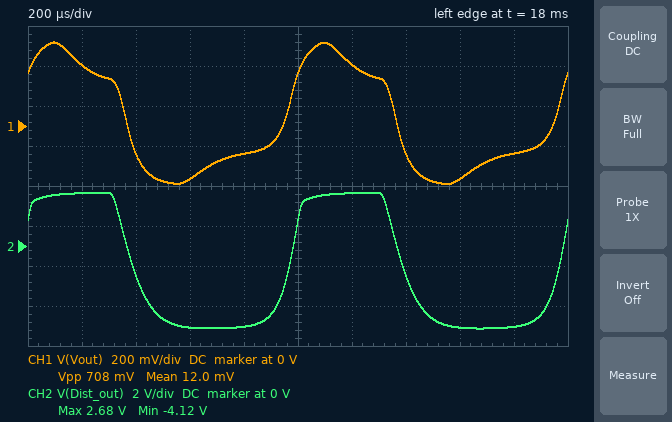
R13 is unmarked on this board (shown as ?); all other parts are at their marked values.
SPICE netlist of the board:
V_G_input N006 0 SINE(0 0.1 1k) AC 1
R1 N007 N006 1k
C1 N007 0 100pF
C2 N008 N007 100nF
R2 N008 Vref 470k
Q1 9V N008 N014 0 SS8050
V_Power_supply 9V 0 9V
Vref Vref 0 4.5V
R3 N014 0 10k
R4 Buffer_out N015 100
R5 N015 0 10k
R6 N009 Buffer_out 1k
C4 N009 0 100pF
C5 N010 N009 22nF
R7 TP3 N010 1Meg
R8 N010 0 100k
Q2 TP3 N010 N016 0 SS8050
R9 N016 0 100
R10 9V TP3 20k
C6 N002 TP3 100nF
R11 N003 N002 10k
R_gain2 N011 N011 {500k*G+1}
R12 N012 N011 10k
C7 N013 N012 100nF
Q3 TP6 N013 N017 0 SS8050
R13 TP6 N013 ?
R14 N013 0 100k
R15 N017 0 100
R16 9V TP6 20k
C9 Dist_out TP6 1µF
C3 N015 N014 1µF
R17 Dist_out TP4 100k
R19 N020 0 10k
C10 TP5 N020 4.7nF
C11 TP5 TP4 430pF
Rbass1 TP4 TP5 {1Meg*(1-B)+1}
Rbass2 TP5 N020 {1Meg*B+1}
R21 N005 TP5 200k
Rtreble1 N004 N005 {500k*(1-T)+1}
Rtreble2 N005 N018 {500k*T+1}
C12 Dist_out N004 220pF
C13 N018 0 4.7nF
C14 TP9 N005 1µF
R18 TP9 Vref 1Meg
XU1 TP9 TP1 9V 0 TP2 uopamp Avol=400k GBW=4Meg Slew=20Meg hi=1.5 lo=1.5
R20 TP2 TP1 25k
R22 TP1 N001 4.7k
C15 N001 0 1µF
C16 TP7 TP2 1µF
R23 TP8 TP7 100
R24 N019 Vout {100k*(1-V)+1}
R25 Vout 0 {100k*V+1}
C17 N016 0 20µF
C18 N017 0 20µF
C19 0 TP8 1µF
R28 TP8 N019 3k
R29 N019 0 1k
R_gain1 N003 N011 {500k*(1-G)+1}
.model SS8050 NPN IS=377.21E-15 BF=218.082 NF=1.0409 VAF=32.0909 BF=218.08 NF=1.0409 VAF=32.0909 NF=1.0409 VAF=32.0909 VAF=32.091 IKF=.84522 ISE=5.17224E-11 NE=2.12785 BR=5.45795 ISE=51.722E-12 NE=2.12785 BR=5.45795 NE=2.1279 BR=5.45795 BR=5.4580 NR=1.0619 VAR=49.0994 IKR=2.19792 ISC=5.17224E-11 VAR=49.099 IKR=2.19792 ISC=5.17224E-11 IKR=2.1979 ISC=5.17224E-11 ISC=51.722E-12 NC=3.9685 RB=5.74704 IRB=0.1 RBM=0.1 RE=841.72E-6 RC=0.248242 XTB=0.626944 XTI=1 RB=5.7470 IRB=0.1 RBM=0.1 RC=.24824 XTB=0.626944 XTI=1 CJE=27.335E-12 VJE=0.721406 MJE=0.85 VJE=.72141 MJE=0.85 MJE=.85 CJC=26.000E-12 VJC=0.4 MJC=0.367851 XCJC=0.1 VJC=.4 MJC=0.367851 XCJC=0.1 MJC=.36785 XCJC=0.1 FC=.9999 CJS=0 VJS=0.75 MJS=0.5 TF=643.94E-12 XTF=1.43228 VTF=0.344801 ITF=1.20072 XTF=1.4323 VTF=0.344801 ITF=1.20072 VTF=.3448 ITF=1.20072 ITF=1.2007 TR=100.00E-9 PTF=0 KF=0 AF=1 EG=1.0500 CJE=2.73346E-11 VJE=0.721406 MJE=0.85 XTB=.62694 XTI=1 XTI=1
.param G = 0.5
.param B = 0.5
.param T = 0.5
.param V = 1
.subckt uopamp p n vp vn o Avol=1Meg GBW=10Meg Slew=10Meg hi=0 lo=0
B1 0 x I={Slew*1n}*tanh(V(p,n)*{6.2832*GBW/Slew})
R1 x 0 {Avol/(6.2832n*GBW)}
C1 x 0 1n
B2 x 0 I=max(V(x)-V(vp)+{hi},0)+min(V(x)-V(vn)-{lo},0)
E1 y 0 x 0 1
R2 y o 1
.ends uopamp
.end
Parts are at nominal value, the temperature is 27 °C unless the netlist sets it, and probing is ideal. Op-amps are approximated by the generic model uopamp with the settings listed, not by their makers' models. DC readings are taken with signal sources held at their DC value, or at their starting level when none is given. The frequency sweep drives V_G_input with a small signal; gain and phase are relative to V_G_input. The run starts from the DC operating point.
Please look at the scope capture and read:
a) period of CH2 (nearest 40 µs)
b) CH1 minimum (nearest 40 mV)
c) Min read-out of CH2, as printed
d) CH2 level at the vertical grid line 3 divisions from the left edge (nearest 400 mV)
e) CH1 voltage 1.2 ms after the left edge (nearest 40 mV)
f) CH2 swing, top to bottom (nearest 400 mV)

1.00 ms
-280 mV
-4.12 V
-4.0 V
320 mV
6.8 V
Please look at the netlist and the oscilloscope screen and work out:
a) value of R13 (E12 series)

820 kΩ
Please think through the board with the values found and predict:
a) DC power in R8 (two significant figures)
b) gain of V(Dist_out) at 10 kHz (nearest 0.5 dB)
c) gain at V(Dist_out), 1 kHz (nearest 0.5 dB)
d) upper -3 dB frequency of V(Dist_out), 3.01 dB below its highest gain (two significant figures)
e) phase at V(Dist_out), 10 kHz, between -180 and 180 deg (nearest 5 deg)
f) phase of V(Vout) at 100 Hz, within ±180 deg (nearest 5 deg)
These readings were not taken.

2.8 µW
40.5 dB
39.5 dB
26 kHz
-20 deg
90 deg
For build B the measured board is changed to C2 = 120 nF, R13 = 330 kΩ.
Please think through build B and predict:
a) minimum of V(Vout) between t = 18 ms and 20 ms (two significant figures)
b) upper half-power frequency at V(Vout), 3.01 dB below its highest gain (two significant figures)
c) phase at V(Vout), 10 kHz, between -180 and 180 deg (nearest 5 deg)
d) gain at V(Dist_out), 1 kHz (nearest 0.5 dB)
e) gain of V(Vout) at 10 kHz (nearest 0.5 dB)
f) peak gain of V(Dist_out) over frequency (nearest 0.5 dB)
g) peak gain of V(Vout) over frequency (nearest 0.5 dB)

-300 mV
6.5 kHz
-75 deg
33.5 dB
12.5 dB
35.0 dB
18.5 dB
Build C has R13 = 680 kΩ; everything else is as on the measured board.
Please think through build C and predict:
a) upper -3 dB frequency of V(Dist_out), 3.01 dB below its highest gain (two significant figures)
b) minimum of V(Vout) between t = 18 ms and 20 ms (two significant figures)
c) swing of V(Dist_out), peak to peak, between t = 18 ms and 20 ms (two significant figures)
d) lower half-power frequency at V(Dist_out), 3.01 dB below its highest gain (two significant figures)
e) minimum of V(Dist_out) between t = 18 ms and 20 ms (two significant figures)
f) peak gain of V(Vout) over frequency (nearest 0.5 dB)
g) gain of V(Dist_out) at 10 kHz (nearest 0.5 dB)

29 kHz
-310 mV
7.0 V
630 Hz
-3.7 V
23.5 dB
39.5 dB
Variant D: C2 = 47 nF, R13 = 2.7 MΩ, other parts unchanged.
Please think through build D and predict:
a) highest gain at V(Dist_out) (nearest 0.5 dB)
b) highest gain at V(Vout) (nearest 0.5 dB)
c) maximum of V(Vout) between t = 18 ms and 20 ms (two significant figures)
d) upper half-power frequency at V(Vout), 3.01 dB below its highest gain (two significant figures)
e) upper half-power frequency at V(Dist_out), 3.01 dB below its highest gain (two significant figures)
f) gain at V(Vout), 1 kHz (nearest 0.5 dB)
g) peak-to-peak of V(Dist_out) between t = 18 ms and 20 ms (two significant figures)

-6.0 dB
-22.5 dB
370 mV
6.1 kHz
170 kHz
-27.0 dB
4.8 V
